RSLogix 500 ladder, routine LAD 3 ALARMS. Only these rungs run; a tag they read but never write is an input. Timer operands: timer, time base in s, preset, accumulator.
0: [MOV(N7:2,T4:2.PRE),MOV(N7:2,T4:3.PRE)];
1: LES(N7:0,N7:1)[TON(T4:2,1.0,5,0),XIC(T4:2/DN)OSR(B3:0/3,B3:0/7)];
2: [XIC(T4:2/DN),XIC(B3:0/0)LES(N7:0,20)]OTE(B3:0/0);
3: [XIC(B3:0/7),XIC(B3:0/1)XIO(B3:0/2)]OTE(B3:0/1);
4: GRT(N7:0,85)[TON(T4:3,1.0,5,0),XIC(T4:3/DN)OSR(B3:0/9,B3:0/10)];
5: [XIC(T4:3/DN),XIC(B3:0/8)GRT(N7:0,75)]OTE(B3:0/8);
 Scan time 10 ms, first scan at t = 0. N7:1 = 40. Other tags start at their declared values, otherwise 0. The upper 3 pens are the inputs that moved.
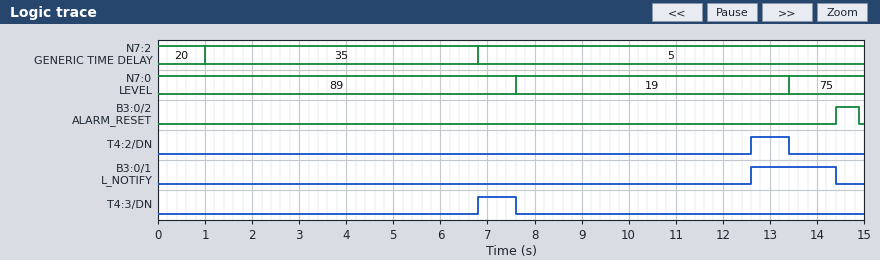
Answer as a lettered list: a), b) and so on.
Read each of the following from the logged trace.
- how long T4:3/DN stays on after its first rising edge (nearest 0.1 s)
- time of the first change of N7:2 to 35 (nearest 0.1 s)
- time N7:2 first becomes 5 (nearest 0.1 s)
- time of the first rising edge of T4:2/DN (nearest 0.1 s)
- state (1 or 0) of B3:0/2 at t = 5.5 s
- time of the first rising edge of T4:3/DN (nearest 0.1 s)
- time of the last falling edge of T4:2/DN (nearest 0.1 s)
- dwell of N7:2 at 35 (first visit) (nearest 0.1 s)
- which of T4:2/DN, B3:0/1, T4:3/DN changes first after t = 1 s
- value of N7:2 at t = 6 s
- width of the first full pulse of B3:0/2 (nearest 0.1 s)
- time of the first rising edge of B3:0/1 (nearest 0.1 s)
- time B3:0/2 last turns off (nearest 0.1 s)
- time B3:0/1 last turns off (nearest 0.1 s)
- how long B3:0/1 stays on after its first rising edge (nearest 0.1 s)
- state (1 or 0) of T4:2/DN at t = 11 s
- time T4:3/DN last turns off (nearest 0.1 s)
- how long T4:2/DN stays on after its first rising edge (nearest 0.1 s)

a) 0.8 s
b) 1.0 s
c) 6.8 s
d) 12.6 s
e) 0
f) 6.8 s
g) 13.4 s
h) 5.8 s
i) T4:3/DN
j) 35
k) 0.5 s
l) 12.6 s
m) 14.9 s
n) 14.4 s
o) 1.8 s
p) 0
q) 7.6 s
r) 0.8 s
